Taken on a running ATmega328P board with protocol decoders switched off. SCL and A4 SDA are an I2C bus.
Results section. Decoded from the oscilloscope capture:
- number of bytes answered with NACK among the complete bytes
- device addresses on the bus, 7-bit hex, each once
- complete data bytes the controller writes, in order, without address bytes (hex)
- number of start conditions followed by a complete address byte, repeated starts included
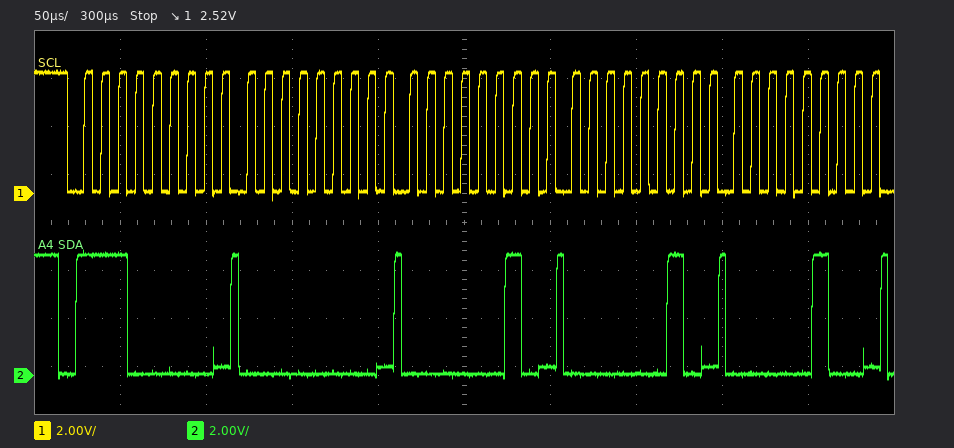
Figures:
0
0x70
00 02 02 04
1
